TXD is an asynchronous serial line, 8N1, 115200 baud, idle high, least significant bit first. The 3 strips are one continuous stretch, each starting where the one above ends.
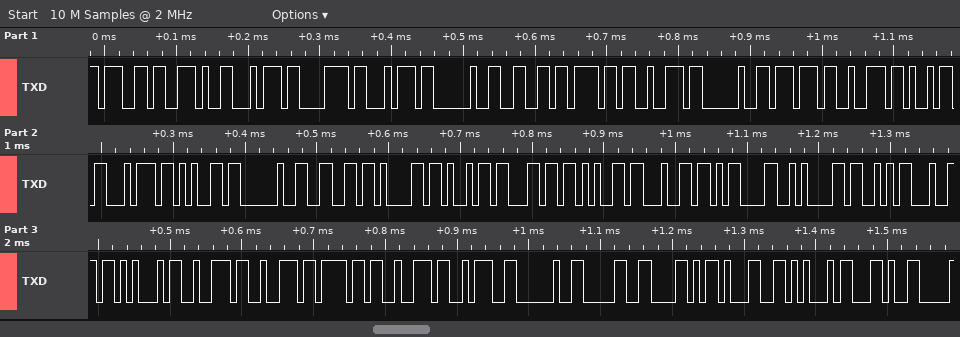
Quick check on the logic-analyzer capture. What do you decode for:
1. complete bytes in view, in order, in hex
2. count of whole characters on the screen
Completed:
67 2E 74 78 74 20 66 6F 72 20 77 72 69 74 65 20 66 61 69 6C 65 64 0D 0A 53 64 45 72 72 6F 72 3A 20 30 58 31 45 2C
38
